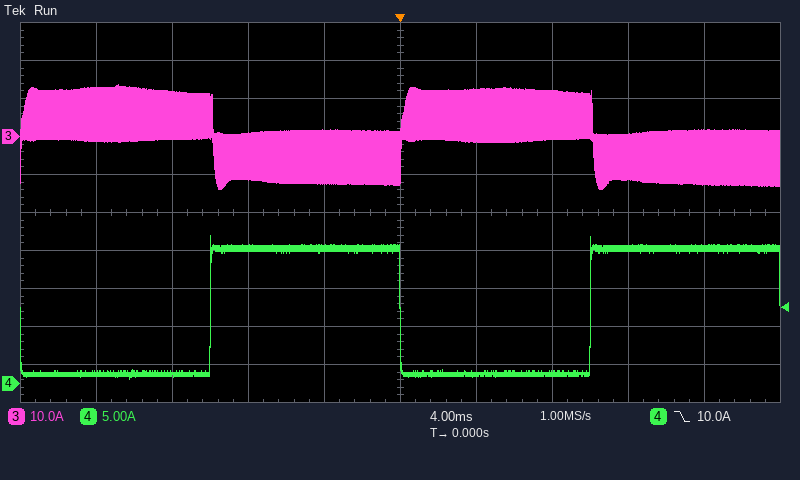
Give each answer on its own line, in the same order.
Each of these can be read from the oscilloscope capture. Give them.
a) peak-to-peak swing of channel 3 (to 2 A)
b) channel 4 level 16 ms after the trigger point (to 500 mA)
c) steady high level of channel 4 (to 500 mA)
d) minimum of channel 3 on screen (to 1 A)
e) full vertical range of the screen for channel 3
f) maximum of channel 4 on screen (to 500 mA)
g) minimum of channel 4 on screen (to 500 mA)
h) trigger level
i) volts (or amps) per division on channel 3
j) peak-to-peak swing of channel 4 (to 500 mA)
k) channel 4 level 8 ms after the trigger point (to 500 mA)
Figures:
28 A
18.0 A
18.0 A
-14 A
100 A
19.5 A
500 mA
10.0 A
10 A
19.0 A
1.5 A
